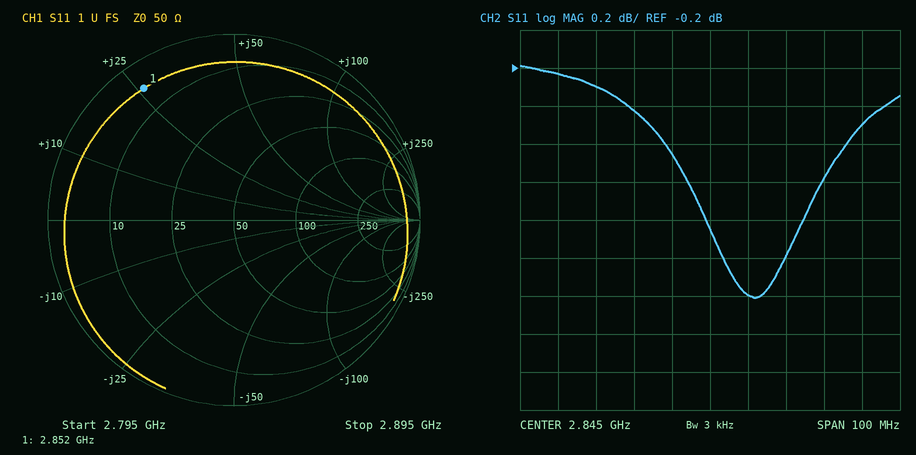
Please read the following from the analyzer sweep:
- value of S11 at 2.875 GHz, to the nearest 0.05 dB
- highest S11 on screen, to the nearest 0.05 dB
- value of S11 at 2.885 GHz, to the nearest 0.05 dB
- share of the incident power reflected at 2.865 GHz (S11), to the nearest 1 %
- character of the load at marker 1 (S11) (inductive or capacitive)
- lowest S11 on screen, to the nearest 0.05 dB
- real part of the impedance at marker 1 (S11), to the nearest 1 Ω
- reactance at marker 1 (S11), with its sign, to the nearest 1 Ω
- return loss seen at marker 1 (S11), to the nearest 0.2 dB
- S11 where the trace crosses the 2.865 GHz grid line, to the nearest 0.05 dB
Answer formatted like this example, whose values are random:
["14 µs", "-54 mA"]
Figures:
["-0.80 dB", "-0.20 dB", "-0.50 dB", "76 %", "inductive", "-1.40 dB", "5 Ω", "+26 Ω", "1.4 dB", "-1.20 dB"]
